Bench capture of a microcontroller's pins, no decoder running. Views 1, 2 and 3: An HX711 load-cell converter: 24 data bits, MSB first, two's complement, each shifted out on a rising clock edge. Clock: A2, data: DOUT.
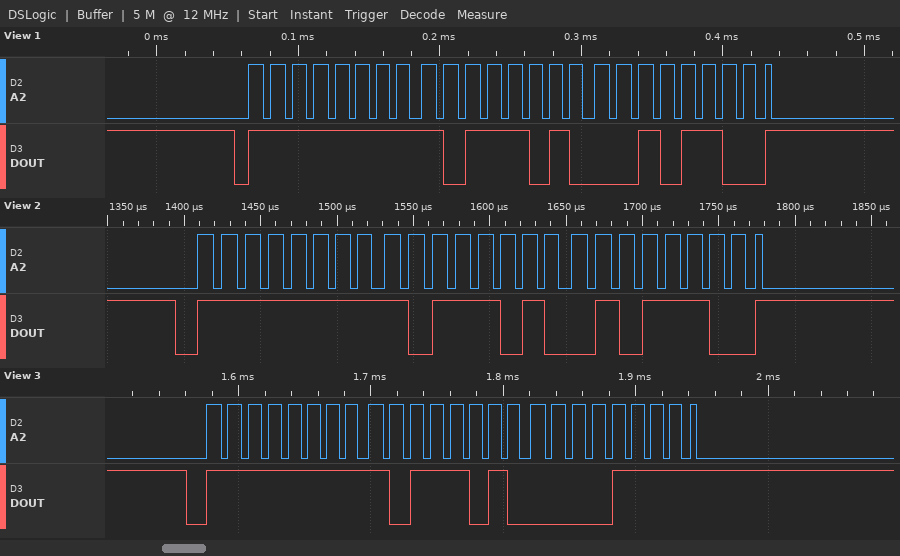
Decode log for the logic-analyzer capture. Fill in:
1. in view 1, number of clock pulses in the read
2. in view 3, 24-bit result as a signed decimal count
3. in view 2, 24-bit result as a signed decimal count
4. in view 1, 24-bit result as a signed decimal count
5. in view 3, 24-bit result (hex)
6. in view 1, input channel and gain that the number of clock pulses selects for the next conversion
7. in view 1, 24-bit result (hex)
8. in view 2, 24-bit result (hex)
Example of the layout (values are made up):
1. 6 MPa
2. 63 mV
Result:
1. 25
2. -17905
3. -17828
4. -17876
5. 0xFFBA0F
6. channel A, gain 128
7. 0xFFBA2C
8. 0xFFBA5C
